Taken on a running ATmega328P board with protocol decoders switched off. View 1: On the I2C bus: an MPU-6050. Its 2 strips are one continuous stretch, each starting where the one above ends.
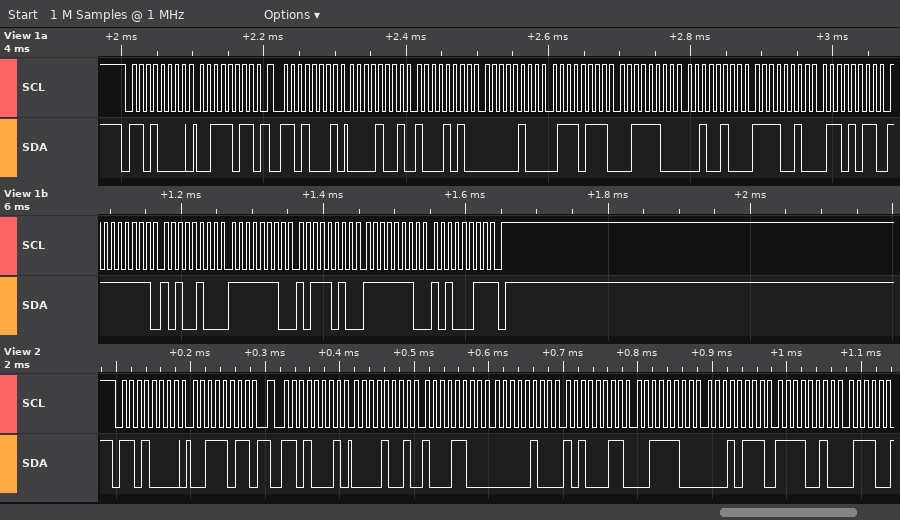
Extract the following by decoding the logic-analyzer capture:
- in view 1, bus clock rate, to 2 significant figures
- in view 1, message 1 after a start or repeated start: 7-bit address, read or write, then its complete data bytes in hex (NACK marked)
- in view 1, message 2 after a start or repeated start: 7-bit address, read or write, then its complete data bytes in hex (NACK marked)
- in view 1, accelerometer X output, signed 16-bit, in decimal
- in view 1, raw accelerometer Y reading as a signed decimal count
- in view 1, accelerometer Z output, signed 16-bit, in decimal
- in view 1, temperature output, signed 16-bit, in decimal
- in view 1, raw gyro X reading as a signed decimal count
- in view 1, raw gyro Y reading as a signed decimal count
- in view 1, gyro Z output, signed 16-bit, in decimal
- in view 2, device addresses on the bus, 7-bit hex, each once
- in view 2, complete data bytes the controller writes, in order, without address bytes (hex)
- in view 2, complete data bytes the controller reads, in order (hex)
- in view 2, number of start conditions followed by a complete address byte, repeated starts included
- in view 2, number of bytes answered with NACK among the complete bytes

100 kHz
0x68 write: 3B
0x68 read: 09 8A 04 77 3C 24 F2 6B FF A4 FE BA FE A3 NACK
2442
1143
15396
-3477
-92
-326
-349
0x68
3B
09 8C 04 A3 3C 17 F2
2
0
